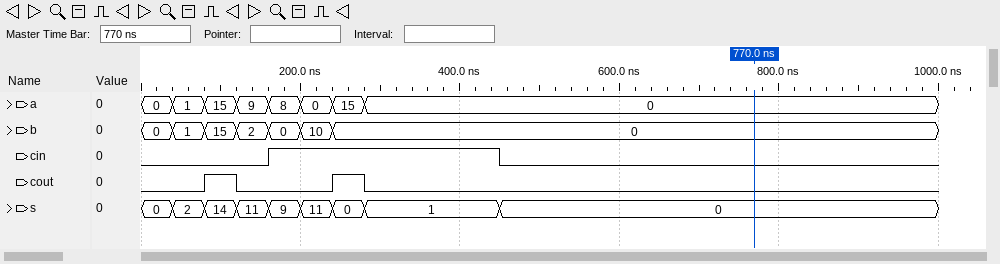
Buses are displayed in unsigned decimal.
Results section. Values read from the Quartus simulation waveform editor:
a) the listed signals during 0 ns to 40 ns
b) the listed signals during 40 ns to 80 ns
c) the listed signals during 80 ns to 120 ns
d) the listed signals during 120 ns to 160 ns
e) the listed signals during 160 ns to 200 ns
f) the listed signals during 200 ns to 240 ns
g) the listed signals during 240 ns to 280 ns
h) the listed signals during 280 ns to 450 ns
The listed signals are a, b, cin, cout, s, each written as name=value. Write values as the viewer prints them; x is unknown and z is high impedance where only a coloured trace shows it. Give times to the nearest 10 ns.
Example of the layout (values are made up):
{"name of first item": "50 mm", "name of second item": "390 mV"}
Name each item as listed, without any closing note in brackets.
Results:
{"the listed signals during 0 ns to 40 ns": "a=0, b=0, cin=0, cout=0, s=0", "the listed signals during 40 ns to 80 ns": "a=1, b=1, cin=0, cout=0, s=2", "the listed signals during 80 ns to 120 ns": "a=15, b=15, cin=0, cout=1, s=14", "the listed signals during 120 ns to 160 ns": "a=9, b=2, cin=0, cout=0, s=11", "the listed signals during 160 ns to 200 ns": "a=8, b=0, cin=1, cout=0, s=9", "the listed signals during 200 ns to 240 ns": "a=0, b=10, cin=1, cout=0, s=11", "the listed signals during 240 ns to 280 ns": "a=15, b=0, cin=1, cout=1, s=0", "the listed signals during 280 ns to 450 ns": "a=0, b=0, cin=1, cout=0, s=1"}
